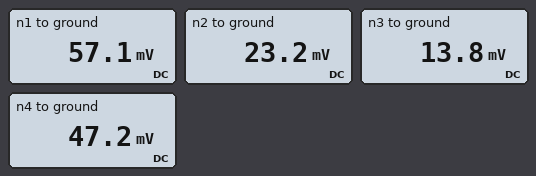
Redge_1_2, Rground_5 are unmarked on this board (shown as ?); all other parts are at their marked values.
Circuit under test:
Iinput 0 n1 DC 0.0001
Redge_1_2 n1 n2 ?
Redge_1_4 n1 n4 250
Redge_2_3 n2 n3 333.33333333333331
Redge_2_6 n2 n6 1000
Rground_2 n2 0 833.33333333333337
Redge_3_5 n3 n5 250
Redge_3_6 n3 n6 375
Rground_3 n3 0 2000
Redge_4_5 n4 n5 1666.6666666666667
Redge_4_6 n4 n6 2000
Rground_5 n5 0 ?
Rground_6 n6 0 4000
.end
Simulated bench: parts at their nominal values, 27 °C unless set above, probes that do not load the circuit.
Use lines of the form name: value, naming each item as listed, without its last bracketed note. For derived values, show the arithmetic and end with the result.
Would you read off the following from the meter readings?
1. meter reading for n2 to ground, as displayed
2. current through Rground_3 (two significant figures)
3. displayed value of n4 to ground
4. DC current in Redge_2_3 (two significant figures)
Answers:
meter reading for n2 to ground, as displayed: 23.2 mV
current through Rground_3: (13.8 mV) / 2 kΩ = 6.9 µA
displayed value of n4 to ground: 47.2 mV
DC current in Redge_2_3: (23.2 mV - 13.8 mV) / 333.3 Ω = 28 µA
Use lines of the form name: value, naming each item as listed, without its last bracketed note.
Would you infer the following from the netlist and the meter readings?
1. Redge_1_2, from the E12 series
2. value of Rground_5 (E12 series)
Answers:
Redge_1_2, from the E12 series: 560 Ω
value of Rground_5: 82 Ω
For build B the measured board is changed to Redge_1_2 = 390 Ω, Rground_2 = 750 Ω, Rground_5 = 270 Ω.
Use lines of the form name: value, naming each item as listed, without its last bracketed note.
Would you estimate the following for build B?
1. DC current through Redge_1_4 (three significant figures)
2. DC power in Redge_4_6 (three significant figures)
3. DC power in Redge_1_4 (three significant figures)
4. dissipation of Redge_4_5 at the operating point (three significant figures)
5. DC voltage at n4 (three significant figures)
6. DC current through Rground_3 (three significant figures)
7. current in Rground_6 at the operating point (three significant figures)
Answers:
DC current through Redge_1_4: 32.0 µA
DC power in Redge_4_6: 270 nW
DC power in Redge_1_4: 255 nW
dissipation of Redge_4_5 at the operating point: 689 nW
DC voltage at n4: 46.6 mV
DC current through Rground_3: 9.70 µA
current in Rground_6 at the operating point: 5.83 µA
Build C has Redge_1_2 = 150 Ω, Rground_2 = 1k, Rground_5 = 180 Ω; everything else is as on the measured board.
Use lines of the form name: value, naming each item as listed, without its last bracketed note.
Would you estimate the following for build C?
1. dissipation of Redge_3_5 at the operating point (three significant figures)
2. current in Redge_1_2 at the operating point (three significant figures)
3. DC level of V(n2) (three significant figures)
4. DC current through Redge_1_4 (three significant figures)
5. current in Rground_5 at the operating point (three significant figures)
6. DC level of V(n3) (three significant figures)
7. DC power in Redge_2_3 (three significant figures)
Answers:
dissipation of Redge_3_5 at the operating point: 347 nW
current in Redge_1_2 at the operating point: 76.6 µA
DC level of V(n2): 31.2 mV
DC current through Redge_1_4: 23.4 µA
current in Rground_5 at the operating point: 53.6 µA
DC level of V(n3): 19.0 mV
DC power in Redge_2_3: 452 nW
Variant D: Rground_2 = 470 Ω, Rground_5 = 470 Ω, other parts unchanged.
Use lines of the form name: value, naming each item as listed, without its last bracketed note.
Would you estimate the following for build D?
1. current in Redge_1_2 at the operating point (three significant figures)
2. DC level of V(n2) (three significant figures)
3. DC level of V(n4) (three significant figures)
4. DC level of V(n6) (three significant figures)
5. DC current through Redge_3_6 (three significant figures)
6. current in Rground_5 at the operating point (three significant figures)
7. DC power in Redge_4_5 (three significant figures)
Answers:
current in Redge_1_2 at the operating point: 64.7 µA
DC level of V(n2): 23.7 mV
DC level of V(n4): 51.2 mV
DC level of V(n6): 22.8 mV
DC current through Redge_3_6: 9.39 µA
current in Rground_5 at the operating point: 34.1 µA
DC power in Redge_4_5: 741 nW
